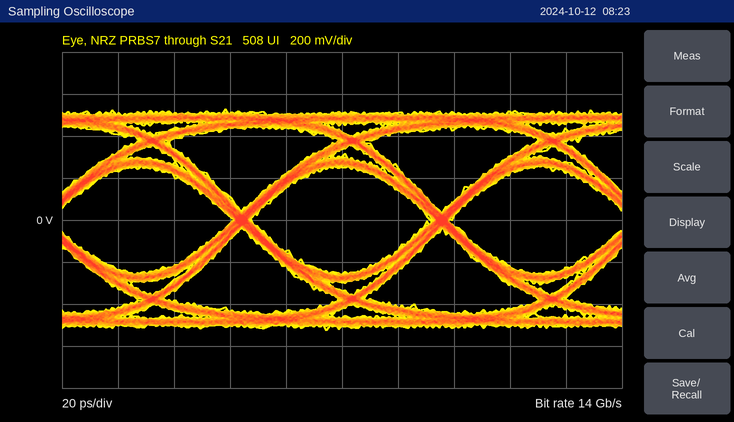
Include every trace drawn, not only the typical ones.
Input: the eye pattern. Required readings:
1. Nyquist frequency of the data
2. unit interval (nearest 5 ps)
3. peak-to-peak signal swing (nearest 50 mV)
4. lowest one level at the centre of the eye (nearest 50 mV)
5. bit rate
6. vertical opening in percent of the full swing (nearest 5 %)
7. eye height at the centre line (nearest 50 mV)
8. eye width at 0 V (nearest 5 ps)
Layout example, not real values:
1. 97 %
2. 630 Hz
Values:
1. 7 GHz
2. 70 ps
3. 1.05 V
4. 250 mV
5. 14 Gb/s
6. 50 %
7. 500 mV
8. 65 ps
